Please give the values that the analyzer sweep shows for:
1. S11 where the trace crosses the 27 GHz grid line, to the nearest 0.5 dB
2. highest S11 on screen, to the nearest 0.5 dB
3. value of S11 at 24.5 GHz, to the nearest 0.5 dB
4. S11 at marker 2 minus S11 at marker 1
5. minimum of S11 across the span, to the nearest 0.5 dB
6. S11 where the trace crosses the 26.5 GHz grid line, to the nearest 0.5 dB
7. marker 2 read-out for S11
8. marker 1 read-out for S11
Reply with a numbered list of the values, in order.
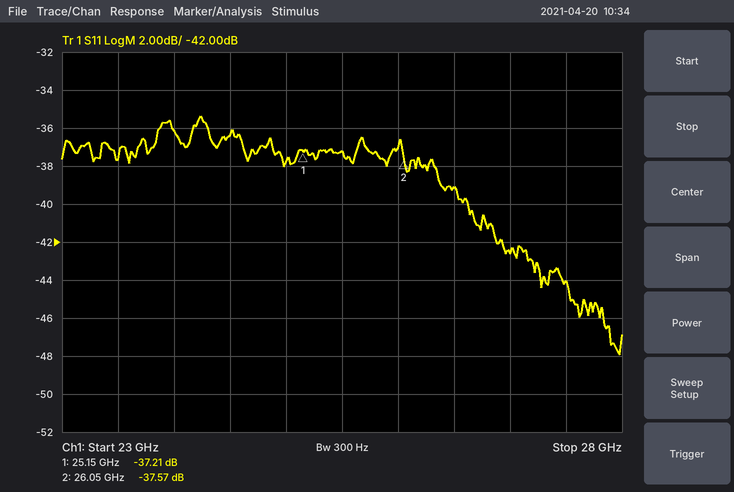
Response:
1. -42.5 dB
2. -35.5 dB
3. -36.5 dB
4. -0.36 dB
5. -48.0 dB
6. -39.0 dB
7. -37.57 dB
8. -37.21 dB
